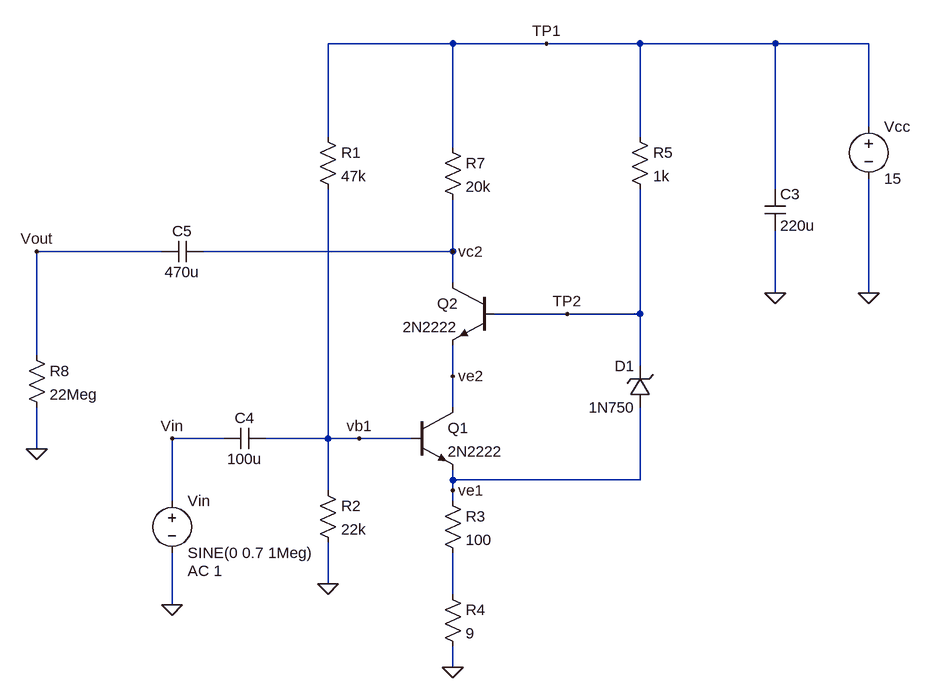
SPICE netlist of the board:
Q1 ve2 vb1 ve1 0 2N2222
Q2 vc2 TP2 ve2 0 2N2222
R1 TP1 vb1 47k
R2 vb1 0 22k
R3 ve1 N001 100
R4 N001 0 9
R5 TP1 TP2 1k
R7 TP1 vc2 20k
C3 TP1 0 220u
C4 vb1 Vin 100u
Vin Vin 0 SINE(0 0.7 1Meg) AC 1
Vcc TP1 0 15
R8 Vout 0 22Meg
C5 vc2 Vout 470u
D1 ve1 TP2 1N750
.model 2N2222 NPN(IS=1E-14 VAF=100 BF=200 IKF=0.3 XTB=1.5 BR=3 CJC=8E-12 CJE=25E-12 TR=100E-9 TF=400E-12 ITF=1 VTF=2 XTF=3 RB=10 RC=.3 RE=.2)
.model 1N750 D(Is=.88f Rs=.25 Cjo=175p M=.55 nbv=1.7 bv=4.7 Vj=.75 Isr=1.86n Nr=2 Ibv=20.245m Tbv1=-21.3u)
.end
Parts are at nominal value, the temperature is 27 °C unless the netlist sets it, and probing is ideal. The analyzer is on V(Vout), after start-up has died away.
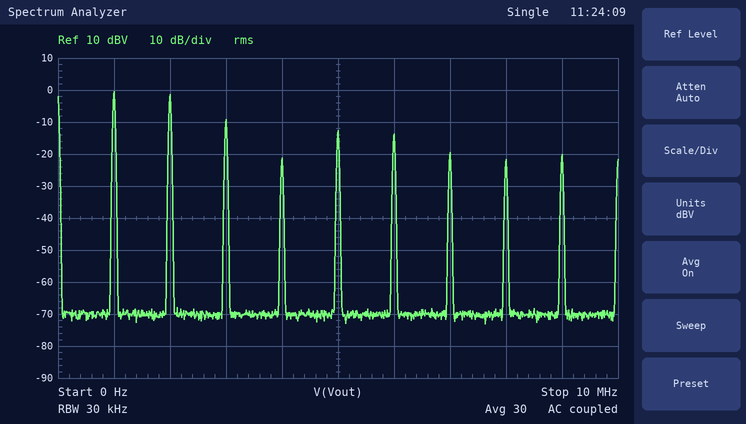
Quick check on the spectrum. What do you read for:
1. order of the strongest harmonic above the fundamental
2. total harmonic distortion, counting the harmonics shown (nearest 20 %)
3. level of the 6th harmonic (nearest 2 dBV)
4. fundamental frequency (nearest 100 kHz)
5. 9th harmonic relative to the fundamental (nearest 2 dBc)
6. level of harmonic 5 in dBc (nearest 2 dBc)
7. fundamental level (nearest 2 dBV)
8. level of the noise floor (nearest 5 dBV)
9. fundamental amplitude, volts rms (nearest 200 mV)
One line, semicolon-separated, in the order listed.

2; 100 %; -14 dBV; 1.0 MHz; -20 dBc; -12 dBc; 0 dBV; -70 dBV; 1.0 V
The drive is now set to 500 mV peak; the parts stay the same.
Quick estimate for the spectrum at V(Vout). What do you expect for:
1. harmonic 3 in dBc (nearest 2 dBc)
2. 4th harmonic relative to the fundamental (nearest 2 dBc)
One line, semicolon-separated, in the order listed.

-8 dBc; -18 dBc
